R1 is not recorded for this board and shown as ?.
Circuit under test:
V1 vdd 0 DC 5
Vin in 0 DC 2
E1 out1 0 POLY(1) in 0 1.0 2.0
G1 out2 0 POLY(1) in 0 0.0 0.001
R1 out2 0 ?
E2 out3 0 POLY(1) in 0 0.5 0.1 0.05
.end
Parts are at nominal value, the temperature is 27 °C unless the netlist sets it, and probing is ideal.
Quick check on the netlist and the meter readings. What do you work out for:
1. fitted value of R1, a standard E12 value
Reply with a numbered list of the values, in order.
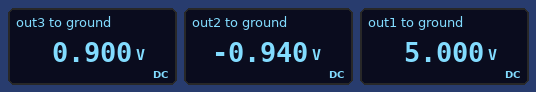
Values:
1. 470 Ω
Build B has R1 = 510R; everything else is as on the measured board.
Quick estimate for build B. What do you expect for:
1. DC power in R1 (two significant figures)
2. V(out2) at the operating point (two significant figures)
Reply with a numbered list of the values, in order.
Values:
1. 2.0 mW
2. -1.0 V
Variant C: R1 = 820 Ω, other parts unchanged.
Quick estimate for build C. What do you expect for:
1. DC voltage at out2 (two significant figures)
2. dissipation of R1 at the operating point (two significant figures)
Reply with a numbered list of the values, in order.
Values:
1. -1.6 V
2. 3.3 mW
